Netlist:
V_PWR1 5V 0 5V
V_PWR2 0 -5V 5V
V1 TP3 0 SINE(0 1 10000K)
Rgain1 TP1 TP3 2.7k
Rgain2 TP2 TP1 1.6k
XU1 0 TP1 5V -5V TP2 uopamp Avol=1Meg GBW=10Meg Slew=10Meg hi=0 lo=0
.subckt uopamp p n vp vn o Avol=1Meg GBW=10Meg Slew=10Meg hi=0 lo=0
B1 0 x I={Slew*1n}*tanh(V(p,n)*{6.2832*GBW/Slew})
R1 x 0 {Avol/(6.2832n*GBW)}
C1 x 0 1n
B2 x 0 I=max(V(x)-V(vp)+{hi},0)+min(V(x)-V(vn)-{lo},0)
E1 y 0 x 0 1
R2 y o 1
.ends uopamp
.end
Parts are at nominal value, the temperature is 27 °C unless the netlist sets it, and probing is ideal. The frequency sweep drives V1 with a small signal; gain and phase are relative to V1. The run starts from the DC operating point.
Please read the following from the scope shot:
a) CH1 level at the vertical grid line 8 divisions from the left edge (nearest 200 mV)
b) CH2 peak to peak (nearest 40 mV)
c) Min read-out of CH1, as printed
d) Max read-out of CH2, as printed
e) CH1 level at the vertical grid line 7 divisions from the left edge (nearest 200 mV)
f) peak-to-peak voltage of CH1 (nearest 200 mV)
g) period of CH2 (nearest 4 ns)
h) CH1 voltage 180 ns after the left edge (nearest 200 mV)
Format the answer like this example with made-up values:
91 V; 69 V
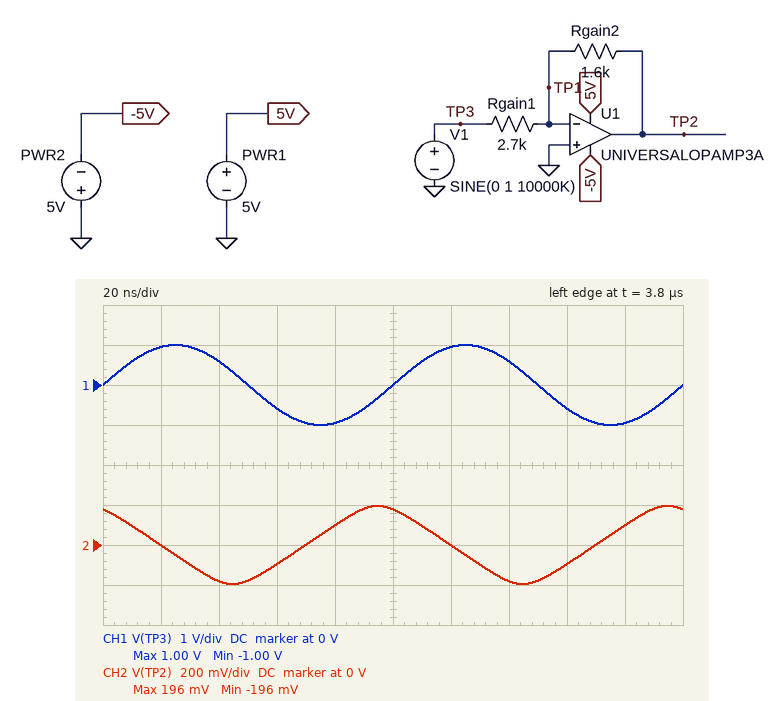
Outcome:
-600 mV; 400 mV; -1.00 V; 196 mV; 600 mV; 2.0 V; 100 ns; -1.0 V
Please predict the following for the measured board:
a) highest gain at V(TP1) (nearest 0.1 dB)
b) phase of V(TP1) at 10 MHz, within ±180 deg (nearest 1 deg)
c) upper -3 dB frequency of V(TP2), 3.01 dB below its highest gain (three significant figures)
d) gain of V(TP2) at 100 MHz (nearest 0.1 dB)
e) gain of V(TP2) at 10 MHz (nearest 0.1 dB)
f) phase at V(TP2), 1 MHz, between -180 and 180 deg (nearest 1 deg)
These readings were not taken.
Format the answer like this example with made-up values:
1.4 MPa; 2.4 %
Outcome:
-8.6 dB; 32 deg; 6.28 MHz; -28.6 dB; -10.0 dB; 171 deg
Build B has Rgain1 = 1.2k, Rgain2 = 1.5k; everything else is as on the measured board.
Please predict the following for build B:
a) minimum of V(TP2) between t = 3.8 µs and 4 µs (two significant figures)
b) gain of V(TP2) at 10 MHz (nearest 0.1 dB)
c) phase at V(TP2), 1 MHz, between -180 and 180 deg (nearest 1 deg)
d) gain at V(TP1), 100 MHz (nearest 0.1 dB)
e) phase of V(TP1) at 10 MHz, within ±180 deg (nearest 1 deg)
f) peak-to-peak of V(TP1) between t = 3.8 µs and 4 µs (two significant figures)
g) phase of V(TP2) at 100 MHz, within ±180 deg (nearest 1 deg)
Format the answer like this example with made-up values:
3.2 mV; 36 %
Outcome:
-220 mV; -5.9 dB; 167 deg; -5.1 dB; 24 deg; 1.1 V; 92 deg
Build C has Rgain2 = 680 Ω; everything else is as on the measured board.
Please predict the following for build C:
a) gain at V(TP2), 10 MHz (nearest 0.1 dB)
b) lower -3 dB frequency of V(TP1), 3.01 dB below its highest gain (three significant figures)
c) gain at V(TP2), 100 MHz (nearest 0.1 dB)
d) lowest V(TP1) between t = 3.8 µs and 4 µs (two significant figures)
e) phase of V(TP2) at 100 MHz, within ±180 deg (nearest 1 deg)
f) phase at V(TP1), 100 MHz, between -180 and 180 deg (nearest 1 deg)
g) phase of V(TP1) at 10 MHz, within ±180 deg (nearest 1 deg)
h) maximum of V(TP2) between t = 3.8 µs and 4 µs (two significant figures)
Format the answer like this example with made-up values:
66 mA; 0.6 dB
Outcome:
-16.1 dB; 7.99 MHz; -34.0 dB; -170 mV; 94 deg; 5 deg; 39 deg; 140 mV
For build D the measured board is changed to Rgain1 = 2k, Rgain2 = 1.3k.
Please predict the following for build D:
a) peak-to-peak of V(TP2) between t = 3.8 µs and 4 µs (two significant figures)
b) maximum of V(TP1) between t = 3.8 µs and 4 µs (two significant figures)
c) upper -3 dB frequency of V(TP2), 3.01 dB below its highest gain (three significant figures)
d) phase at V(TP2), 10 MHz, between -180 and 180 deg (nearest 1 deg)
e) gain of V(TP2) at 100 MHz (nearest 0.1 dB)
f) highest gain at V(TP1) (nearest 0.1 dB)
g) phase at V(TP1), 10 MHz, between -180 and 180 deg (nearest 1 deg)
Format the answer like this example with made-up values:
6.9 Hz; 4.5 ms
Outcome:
400 mV; 380 mV; 6.06 MHz; 121 deg; -28.1 dB; -8.1 dB; 31 deg
